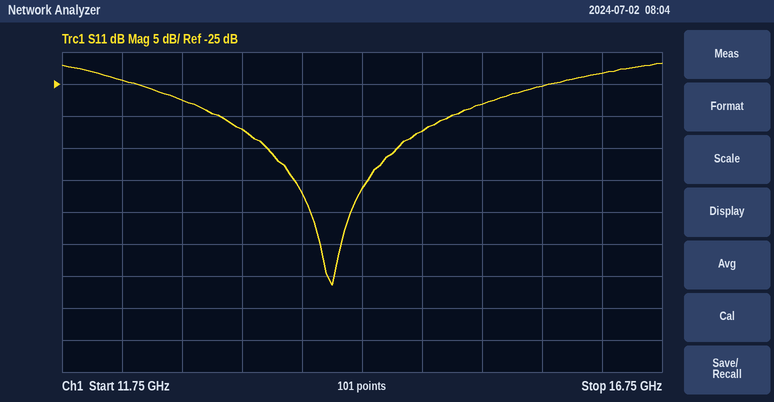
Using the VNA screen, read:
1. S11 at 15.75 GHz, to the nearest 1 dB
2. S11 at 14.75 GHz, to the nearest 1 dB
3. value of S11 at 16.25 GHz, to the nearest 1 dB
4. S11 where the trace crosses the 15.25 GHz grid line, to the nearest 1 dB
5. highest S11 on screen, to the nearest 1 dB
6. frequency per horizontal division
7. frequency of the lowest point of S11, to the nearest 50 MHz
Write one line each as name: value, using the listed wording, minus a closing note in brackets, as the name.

S11 at 15.75 GHz, to the nearest 1 dB: -25 dB
S11 at 14.75 GHz, to the nearest 1 dB: -32 dB
value of S11 at 16.25 GHz, to the nearest 1 dB: -23 dB
S11 where the trace crosses the 15.25 GHz grid line, to the nearest 1 dB: -28 dB
highest S11 on screen, to the nearest 1 dB: -22 dB
frequency per horizontal division: 500 MHz
frequency of the lowest point of S11, to the nearest 50 MHz: 14.00 GHz
